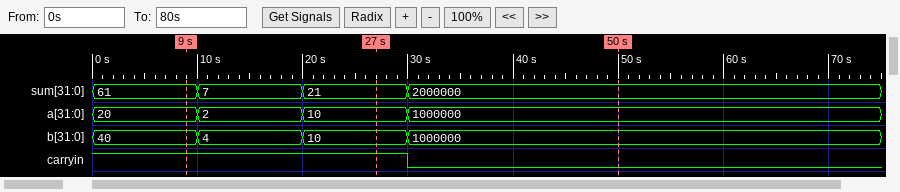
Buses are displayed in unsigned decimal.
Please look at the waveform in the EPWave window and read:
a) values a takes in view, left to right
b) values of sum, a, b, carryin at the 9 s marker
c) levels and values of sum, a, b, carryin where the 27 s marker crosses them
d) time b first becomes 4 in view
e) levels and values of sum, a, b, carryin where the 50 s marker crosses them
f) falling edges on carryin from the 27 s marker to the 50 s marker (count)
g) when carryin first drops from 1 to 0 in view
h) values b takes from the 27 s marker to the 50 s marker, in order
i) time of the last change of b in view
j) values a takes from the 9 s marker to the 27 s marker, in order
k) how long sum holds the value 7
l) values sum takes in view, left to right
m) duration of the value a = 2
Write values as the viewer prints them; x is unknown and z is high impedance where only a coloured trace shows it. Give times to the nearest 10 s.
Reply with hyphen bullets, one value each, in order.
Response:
- 20, 2, 10, 1000000
- sum=61, a=20, b=40, carryin=1
- sum=21, a=10, b=10, carryin=1
- 10 s
- sum=2000000, a=1000000, b=1000000, carryin=0
- 1
- 30 s
- 10, 1000000
- 30 s
- 20, 2, 10
- 10 s
- 61, 7, 21, 2000000
- 10 s
